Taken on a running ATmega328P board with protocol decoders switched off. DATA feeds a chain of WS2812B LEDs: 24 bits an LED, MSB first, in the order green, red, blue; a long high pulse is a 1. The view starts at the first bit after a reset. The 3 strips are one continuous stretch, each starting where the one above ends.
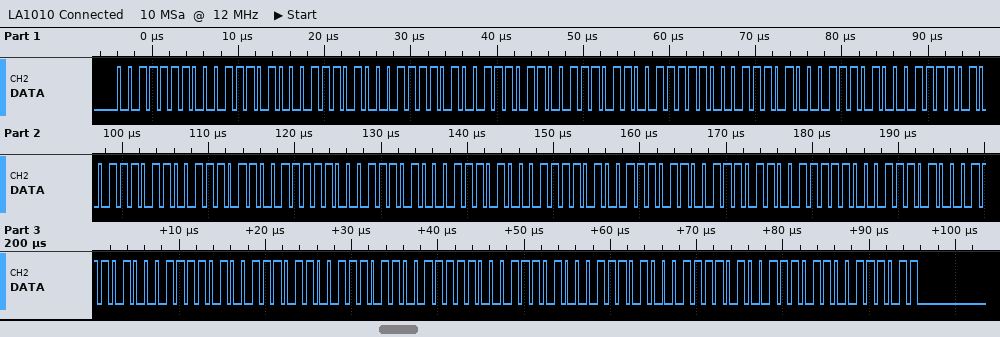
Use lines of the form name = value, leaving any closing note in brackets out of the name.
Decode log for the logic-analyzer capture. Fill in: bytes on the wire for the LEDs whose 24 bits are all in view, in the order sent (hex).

bytes on the wire for the LEDs whose 24 bits are all in view, in the order sent = 3E 3A 3A 3D 3B 3B 3E 3A 3A 3D 3B 3B 3E 3A 3A 3D 3B 3B 3E 3A 3A 3D 3B 3B 3E 3A 3A 3D 3B 3B
